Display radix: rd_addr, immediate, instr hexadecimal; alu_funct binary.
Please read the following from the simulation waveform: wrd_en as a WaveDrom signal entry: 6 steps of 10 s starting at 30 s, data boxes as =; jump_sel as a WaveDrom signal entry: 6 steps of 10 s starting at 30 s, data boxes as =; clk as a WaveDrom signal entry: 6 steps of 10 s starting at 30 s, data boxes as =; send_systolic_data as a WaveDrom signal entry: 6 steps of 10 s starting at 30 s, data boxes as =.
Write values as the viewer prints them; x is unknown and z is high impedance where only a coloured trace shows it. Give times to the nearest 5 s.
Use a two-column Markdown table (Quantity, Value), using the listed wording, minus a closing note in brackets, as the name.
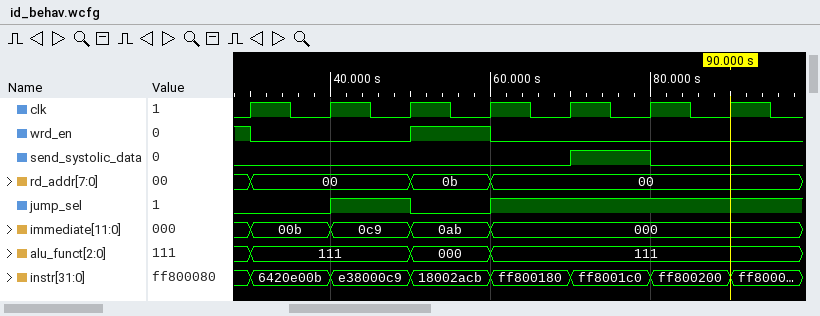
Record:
| Quantity | Value |
|---|---|
| wrd_en as a WaveDrom signal entry: 6 steps of 10 s starting at 30 s, data boxes as = | {name: 'wrd_en', wave: '0.10..'} |
| jump_sel as a WaveDrom signal entry: 6 steps of 10 s starting at 30 s, data boxes as = | {name: 'jump_sel', wave: '0101..'} |
| clk as a WaveDrom signal entry: 6 steps of 10 s starting at 30 s, data boxes as = | {name: 'clk', wave: 'p.....'} |
| send_systolic_data as a WaveDrom signal entry: 6 steps of 10 s starting at 30 s, data boxes as = | {name: 'send_systolic_data', wave: '0...10'} |
